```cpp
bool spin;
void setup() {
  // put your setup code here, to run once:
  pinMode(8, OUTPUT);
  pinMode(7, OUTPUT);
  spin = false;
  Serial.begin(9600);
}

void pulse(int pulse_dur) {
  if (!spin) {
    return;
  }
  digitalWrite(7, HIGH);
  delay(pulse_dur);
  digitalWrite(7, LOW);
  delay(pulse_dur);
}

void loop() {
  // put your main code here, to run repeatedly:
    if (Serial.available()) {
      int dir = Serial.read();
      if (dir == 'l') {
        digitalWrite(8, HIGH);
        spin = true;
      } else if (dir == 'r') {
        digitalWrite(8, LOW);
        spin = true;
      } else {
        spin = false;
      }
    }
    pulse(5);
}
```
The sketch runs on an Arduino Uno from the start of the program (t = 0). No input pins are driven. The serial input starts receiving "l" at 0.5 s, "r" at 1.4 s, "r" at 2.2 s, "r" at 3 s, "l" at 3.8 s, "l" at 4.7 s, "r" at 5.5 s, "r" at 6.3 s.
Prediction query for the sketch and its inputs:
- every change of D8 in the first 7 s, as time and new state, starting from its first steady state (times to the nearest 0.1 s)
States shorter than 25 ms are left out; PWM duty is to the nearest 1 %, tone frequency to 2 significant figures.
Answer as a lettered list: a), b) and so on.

a) 0 s low; 0.5 s high; 1.4 s low; 3.8 s high; 5.5 s low
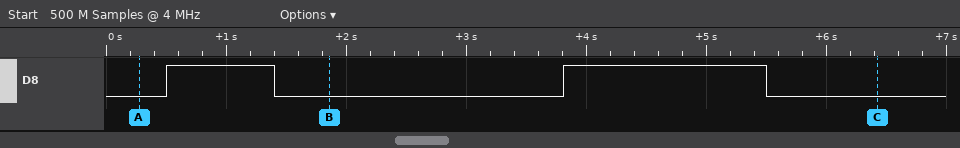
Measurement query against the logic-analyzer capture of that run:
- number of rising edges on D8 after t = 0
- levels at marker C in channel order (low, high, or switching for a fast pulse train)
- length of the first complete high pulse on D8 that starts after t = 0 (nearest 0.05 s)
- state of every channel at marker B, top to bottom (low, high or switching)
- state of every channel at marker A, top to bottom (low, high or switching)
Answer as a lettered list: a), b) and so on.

a) 2
b) D8 low
c) 0.90 s
d) D8 low
e) D8 low
